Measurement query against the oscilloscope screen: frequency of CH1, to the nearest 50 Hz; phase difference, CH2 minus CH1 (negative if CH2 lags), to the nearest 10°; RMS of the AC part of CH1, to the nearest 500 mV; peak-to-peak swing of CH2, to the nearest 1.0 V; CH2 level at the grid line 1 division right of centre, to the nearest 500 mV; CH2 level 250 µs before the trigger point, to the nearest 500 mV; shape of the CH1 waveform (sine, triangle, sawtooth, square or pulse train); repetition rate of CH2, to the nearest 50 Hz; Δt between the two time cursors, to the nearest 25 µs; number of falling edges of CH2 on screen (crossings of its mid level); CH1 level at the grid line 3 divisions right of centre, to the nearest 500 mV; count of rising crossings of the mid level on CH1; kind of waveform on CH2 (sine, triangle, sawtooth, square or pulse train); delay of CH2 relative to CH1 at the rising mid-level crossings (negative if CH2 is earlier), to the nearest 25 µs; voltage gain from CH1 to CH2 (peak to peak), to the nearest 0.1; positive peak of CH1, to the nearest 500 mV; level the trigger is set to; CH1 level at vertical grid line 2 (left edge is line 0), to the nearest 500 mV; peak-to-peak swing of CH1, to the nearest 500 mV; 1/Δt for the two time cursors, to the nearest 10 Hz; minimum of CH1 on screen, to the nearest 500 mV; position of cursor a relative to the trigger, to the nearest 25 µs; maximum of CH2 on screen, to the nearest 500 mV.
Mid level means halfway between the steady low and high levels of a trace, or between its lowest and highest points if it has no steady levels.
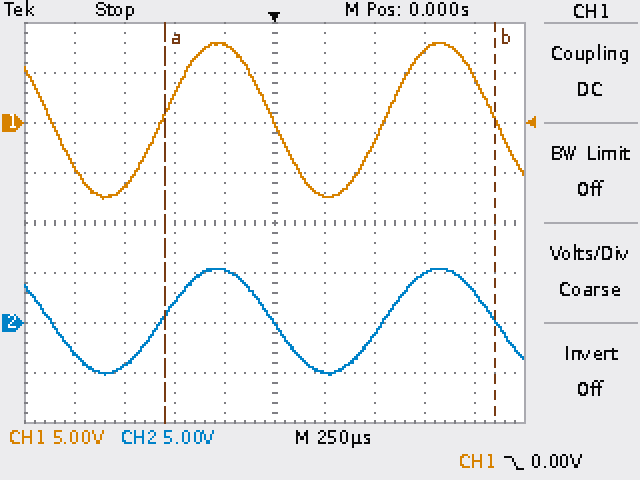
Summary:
900 Hz
0°
5.5 V
11.0 V
-5.0 V
5.5 V
sine
900 Hz
1.650 ms
3
7.0 V
2
sine
0 µs
0.7
8.0 V
0.00 V
-6.5 V
15.5 V
610 Hz
-7.5 V
-550 µs
5.5 V
